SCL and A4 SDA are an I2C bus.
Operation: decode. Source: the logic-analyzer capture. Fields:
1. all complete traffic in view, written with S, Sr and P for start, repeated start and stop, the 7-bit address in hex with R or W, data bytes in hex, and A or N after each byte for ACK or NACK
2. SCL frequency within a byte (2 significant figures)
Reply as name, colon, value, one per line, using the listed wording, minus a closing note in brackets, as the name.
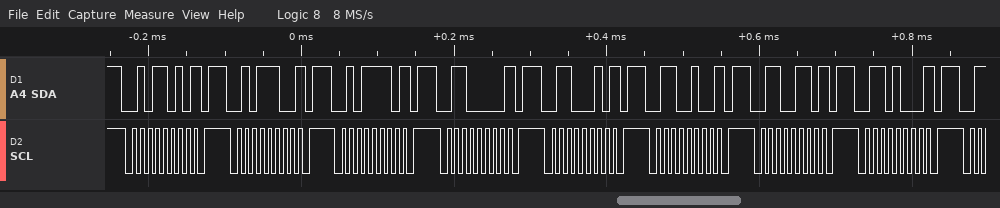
all complete traffic in view, written with S, Sr and P for start, repeated start and stop, the 7-bit address in hex with R or W, data bytes in hex, and A or N after each byte for ACK or NACK: S 2DW N P S 2EW N P S 2FW N P S 30W N P S 31W N P S 32W N P S 33W N P S 34W N P
SCL frequency within a byte: 100 kHz
